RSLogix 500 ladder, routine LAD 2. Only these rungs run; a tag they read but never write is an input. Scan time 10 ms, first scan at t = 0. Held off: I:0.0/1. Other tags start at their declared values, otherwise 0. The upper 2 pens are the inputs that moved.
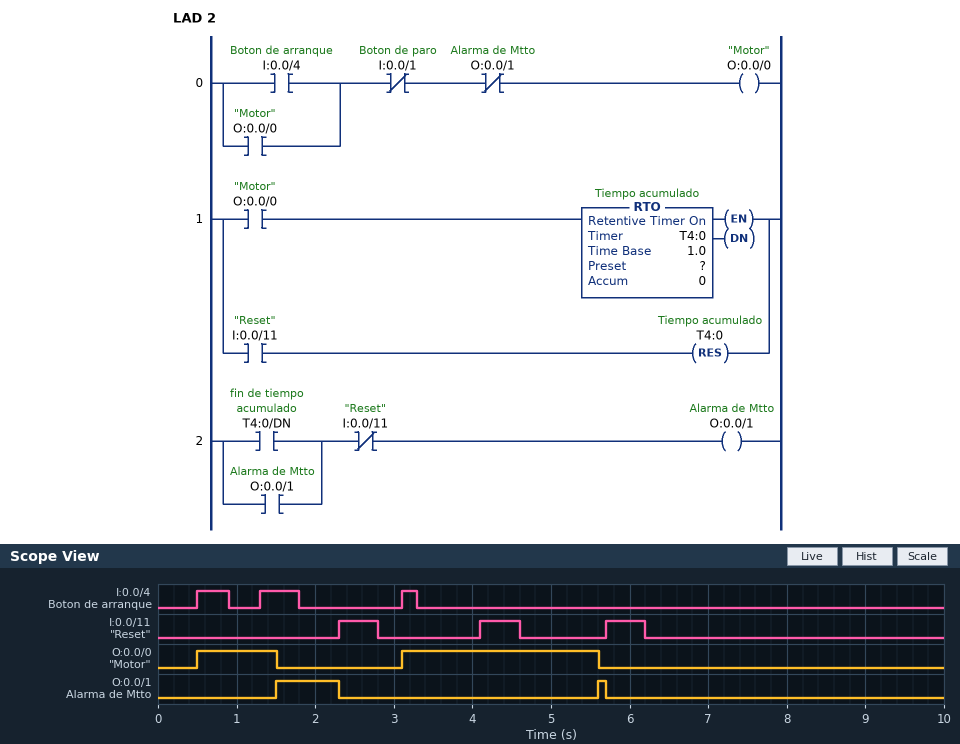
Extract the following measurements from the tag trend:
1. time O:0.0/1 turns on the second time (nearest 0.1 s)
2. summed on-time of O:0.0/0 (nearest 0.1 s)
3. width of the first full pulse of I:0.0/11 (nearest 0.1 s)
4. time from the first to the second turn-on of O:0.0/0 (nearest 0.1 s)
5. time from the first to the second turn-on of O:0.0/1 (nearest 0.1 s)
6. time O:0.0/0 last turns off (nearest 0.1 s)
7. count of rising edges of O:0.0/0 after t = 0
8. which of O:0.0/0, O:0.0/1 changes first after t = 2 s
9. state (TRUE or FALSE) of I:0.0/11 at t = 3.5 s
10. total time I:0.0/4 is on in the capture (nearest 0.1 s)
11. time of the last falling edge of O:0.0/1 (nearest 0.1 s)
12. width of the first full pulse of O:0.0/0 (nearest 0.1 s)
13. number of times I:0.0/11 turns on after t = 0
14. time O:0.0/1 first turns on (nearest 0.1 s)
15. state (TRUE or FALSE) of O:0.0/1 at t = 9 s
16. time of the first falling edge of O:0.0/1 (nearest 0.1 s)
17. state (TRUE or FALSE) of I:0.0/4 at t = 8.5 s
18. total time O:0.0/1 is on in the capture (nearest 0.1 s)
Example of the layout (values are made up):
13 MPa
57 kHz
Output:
5.6 s
3.5 s
0.5 s
2.6 s
4.1 s
5.6 s
2
O:0.0/1
FALSE
1.1 s
5.7 s
1.0 s
3
1.5 s
FALSE
2.3 s
FALSE
0.9 s
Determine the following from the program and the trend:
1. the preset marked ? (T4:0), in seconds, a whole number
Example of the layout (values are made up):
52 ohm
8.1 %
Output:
1 s
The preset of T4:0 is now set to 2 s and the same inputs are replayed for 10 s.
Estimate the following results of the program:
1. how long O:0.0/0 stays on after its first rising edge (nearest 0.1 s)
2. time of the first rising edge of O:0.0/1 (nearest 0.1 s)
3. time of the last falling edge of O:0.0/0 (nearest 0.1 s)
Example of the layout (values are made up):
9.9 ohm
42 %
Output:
7.7 s
8.2 s
8.2 s
